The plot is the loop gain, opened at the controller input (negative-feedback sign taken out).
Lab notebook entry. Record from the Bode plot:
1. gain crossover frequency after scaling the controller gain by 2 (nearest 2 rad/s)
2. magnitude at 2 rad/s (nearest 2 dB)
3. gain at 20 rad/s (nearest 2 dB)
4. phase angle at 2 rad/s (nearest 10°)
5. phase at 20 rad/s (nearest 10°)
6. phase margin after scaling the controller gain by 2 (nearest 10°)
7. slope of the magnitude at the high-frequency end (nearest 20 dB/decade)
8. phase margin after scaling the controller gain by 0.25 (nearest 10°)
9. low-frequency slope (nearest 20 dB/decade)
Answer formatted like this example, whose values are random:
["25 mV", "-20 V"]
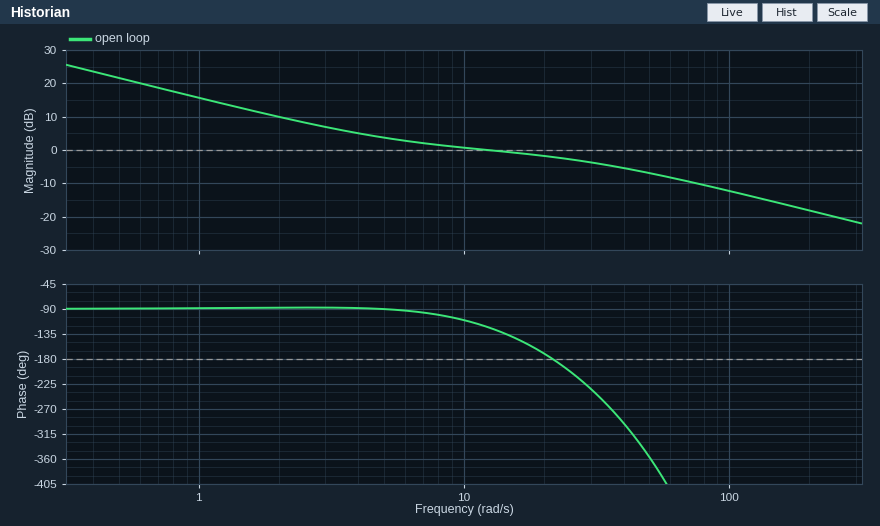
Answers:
["44 rad/s", "10 dB", "-2 dB", "-90°", "-170°", "-140°", "-20 dB/decade", "90°", "-20 dB/decade"]
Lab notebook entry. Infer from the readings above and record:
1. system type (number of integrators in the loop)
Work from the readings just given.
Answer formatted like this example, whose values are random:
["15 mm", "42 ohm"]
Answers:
["1"]
